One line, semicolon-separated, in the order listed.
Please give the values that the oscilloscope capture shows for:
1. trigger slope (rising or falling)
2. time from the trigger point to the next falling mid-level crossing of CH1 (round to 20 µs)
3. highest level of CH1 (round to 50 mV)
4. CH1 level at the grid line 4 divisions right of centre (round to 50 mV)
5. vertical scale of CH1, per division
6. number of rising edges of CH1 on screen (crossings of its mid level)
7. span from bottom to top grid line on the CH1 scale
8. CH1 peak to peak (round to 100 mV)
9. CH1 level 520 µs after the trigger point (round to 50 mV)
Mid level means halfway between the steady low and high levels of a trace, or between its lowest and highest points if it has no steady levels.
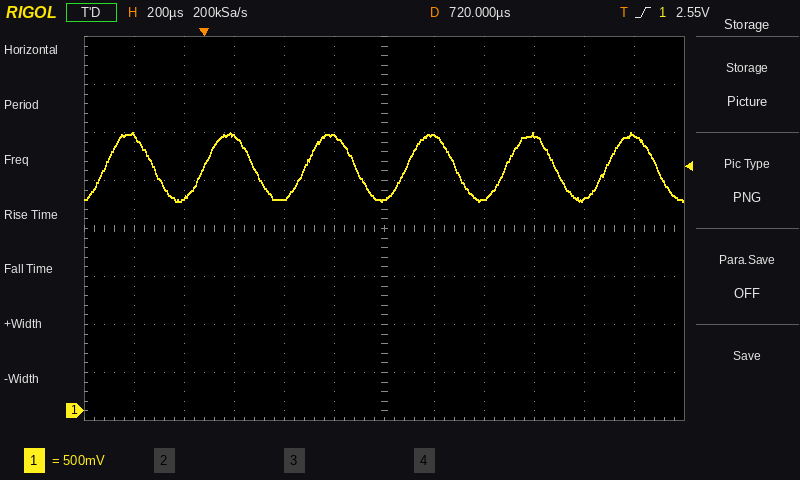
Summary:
rising; 200 µs; 2.90 V; 2.20 V; 500 mV; 6; 4 V; 700 mV; 2.85 V
